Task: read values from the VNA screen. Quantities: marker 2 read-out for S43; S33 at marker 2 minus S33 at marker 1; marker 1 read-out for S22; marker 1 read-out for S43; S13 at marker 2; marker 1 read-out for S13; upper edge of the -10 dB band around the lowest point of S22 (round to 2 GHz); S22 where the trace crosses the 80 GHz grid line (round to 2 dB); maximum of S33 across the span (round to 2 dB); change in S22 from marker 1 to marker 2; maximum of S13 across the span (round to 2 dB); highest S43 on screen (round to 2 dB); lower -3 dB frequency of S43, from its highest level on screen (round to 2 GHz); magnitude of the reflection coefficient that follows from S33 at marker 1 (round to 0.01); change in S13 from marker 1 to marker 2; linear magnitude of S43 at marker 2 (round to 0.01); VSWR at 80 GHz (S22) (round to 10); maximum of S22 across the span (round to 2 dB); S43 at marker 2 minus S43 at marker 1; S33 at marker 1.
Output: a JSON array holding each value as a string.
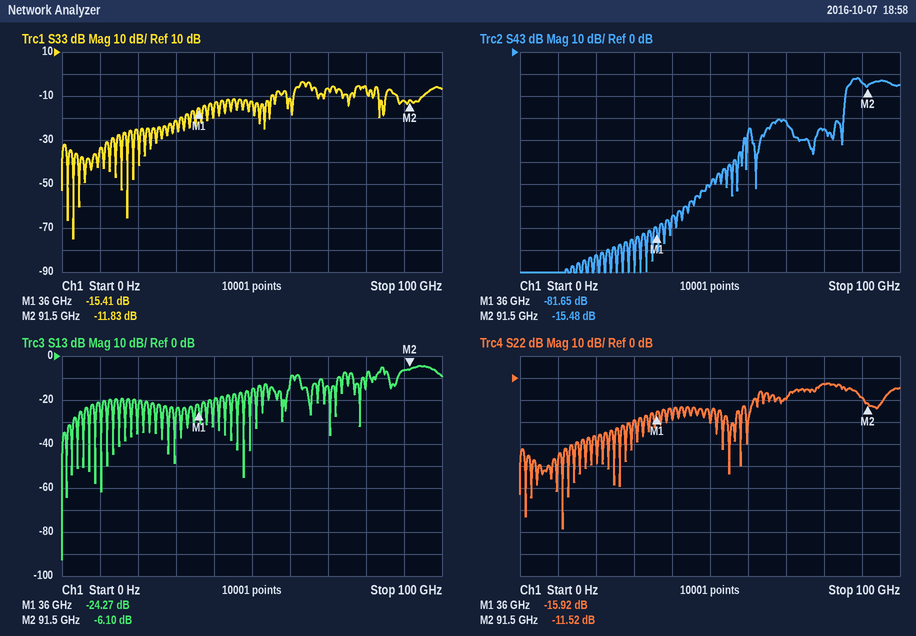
["-15.48 dB", "3.58 dB", "-15.92 dB", "-81.65 dB", "-6.10 dB", "-24.27 dB", "62 GHz", "-2 dB", "-4 dB", "4.40 dB", "-4 dB", "-12 dB", "86 GHz", "0.17", "18.17 dB", "0.17", "10", "-2 dB", "66.17 dB", "-15.41 dB"]
